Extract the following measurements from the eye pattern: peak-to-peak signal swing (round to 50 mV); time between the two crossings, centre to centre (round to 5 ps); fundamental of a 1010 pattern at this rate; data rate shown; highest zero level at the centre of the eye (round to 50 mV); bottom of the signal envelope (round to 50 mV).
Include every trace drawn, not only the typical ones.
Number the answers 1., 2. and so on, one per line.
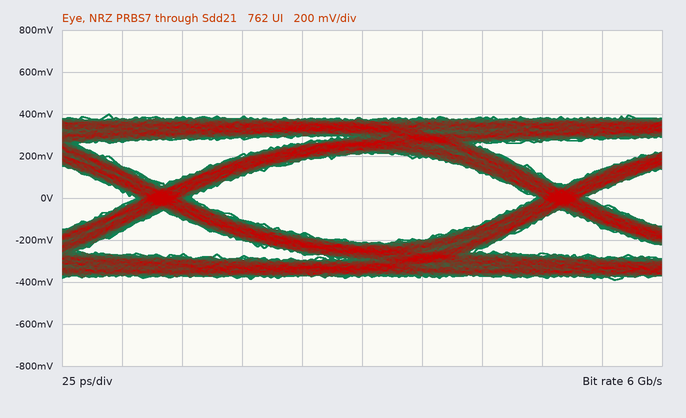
1. 800 mV
2. 165 ps
3. 3 GHz
4. 6 Gb/s
5. -200 mV
6. -400 mV
